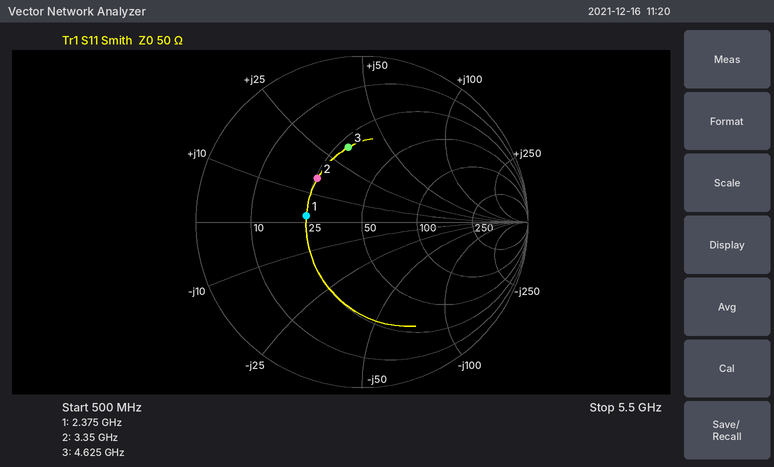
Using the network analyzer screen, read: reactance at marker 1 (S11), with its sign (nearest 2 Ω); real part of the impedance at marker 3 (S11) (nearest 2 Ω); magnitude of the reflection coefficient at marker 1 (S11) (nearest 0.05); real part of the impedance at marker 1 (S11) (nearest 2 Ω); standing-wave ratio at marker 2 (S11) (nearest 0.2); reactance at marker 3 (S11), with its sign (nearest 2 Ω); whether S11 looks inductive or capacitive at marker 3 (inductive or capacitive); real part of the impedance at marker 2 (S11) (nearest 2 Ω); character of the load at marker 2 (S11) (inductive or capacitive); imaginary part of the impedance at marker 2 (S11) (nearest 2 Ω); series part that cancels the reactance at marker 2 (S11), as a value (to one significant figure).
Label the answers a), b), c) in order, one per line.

a) +2 Ω
b) 28 Ω
c) 0.35
d) 24 Ω
e) 2.2
f) +32 Ω
g) inductive
h) 26 Ω
i) inductive
j) +16 Ω
k) 3 pF
